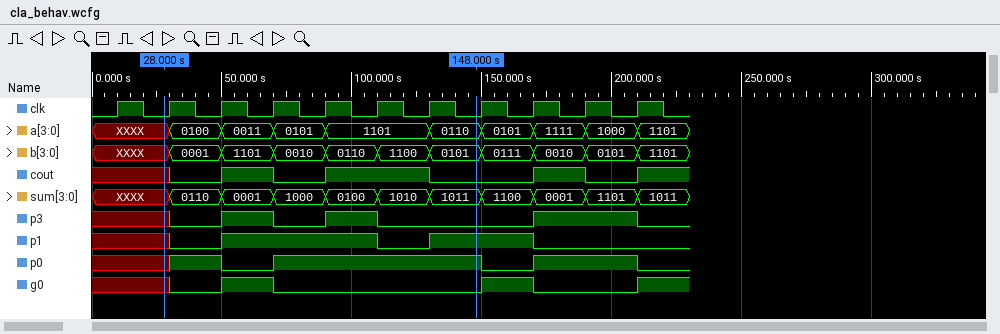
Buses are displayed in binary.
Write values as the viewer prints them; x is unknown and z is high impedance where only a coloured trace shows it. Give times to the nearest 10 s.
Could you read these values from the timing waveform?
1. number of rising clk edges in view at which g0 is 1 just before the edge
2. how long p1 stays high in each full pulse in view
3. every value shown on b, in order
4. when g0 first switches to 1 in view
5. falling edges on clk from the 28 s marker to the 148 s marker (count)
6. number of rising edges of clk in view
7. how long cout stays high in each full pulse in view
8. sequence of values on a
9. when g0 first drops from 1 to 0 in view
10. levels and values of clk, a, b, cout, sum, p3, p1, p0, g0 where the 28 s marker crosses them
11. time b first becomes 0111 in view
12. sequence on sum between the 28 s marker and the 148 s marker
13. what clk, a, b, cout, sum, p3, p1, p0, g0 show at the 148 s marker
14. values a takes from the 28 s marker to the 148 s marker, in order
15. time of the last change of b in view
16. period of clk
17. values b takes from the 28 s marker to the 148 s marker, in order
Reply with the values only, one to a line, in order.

2
60 s, 40 s
XXXX, 0001, 1101, 0010, 0110, 1100, 0101, 0111, 0010, 0101, 1101
50 s
6
11
20 s, 40 s, 20 s
XXXX, 0100, 0011, 0101, 1101, 0110, 0101, 1111, 1000, 1101
70 s
clk=0, a=XXXX, b=XXXX, cout=x, sum=XXXX, p3=x, p1=x, p0=x, g0=x
150 s
XXXX, 0110, 0001, 1000, 0100, 1010, 1011
clk=0, a=0110, b=0101, cout=0, sum=1011, p3=0, p1=1, p0=1, g0=0
XXXX, 0100, 0011, 0101, 1101, 0110
210 s
20 s
XXXX, 0001, 1101, 0010, 0110, 1100, 0101
